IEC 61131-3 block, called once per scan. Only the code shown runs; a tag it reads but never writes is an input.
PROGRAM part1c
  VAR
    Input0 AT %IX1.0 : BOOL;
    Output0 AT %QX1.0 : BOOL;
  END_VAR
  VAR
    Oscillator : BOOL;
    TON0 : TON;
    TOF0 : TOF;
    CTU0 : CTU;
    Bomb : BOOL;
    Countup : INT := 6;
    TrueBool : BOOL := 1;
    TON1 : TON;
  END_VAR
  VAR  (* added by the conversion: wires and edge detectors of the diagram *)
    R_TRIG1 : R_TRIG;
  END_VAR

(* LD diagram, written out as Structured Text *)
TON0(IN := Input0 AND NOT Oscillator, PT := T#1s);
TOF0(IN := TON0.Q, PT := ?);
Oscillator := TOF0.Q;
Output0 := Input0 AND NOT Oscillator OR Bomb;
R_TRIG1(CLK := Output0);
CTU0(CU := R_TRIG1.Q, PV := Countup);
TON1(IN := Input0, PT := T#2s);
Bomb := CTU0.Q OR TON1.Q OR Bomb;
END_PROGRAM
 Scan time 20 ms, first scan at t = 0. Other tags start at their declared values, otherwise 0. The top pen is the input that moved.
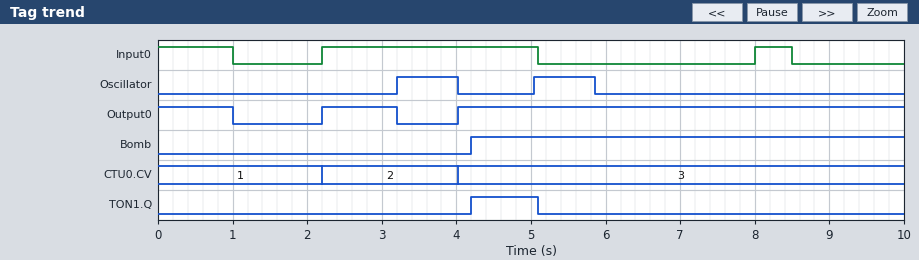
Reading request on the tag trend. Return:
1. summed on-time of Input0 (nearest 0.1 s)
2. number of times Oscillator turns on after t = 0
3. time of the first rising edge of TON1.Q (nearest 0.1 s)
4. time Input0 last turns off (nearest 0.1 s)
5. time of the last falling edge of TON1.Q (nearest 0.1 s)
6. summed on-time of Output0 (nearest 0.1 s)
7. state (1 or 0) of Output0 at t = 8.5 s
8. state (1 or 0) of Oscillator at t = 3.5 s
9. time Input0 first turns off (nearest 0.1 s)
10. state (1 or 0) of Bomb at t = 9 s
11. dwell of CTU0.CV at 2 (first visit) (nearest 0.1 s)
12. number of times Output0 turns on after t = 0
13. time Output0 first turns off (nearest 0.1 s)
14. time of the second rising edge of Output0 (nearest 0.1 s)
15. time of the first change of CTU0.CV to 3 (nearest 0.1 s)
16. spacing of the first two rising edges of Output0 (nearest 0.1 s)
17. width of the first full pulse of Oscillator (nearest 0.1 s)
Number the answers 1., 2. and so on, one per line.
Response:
1. 4.4 s
2. 2
3. 4.2 s
4. 8.5 s
5. 5.1 s
6. 8.0 s
7. 1
8. 1
9. 1.0 s
10. 1
11. 1.8 s
12. 2
13. 1.0 s
14. 4.0 s
15. 4.0 s
16. 1.8 s
17. 0.8 s
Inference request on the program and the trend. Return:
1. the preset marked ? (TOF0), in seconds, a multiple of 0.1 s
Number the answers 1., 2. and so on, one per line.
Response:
1. 0.8 s
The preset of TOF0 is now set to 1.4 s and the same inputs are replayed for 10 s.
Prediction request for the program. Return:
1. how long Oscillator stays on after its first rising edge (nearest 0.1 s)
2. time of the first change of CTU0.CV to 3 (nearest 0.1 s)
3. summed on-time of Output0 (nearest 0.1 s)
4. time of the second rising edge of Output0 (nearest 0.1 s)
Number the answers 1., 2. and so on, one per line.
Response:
1. 1.4 s
2. 4.2 s
3. 7.8 s
4. 4.2 s
